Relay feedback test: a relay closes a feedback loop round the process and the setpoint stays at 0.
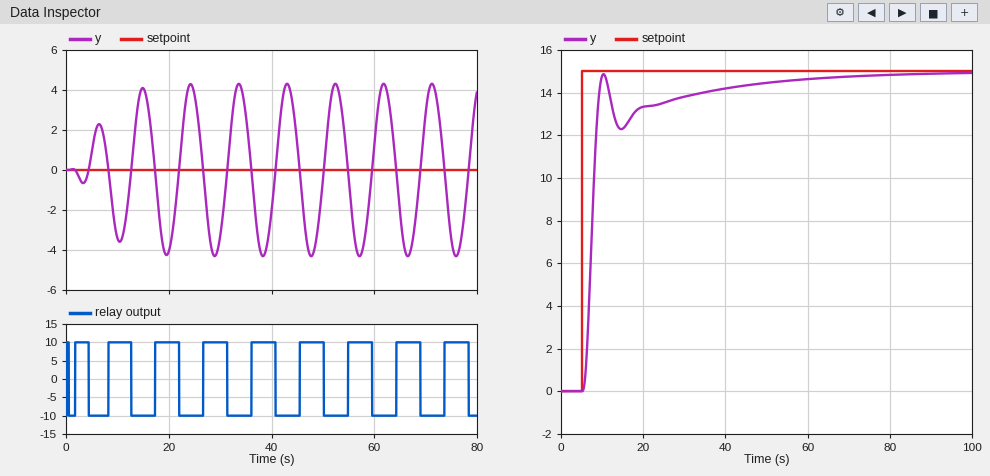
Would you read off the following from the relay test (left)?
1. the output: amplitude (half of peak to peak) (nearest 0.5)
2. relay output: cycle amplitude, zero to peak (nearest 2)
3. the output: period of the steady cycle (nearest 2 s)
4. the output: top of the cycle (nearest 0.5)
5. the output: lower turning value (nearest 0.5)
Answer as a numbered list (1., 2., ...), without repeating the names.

1. 4.5
2. 10
3. 10 s
4. 4.5
5. -4.5
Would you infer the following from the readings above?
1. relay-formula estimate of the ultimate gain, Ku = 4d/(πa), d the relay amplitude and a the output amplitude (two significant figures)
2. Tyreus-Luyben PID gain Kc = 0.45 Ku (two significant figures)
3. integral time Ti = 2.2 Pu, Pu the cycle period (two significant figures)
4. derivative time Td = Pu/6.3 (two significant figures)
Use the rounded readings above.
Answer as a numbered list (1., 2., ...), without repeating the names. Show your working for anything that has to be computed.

1. 4 × 10 / (π × 4.5) = 2.8
2. 0.45 × 2.8 = 1.3
3. 2.2 × 10 = 22 s
4. 10 / 6.3 = 1.6 s
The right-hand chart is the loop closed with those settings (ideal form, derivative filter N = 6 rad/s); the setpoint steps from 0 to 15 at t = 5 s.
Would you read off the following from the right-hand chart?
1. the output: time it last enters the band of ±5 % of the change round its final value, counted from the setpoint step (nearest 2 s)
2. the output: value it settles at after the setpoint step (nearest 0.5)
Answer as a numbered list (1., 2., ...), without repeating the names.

1. 36 s
2. 15.0
